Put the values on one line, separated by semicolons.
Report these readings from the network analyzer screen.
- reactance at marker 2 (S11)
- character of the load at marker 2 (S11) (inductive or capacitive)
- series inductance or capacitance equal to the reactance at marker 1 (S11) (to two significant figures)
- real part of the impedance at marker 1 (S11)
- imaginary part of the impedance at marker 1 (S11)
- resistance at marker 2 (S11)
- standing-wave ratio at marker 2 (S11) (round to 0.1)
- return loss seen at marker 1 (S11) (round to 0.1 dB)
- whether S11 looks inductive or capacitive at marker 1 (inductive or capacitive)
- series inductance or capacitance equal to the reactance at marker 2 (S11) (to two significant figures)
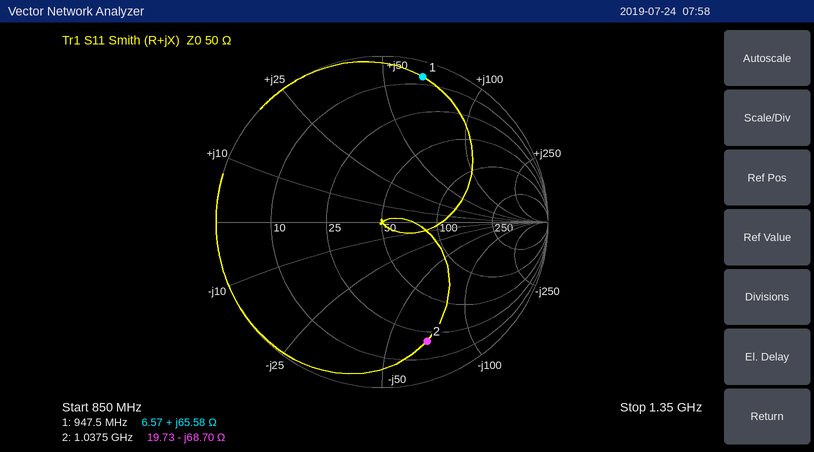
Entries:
-68.70 Ω; capacitive; 11 nH; 6.57 Ω; +65.58 Ω; 19.73 Ω; 7.6; 0.8 dB; inductive; 2.2 pF
